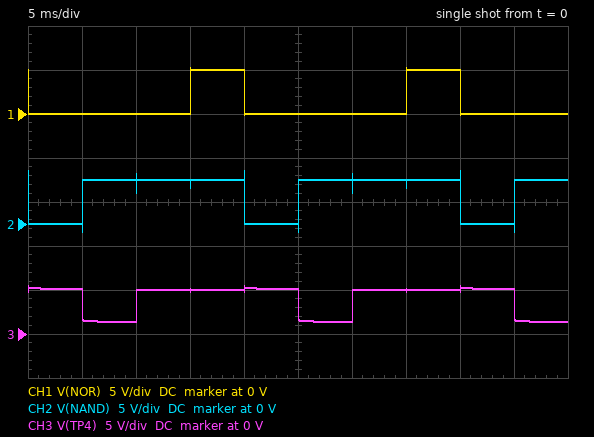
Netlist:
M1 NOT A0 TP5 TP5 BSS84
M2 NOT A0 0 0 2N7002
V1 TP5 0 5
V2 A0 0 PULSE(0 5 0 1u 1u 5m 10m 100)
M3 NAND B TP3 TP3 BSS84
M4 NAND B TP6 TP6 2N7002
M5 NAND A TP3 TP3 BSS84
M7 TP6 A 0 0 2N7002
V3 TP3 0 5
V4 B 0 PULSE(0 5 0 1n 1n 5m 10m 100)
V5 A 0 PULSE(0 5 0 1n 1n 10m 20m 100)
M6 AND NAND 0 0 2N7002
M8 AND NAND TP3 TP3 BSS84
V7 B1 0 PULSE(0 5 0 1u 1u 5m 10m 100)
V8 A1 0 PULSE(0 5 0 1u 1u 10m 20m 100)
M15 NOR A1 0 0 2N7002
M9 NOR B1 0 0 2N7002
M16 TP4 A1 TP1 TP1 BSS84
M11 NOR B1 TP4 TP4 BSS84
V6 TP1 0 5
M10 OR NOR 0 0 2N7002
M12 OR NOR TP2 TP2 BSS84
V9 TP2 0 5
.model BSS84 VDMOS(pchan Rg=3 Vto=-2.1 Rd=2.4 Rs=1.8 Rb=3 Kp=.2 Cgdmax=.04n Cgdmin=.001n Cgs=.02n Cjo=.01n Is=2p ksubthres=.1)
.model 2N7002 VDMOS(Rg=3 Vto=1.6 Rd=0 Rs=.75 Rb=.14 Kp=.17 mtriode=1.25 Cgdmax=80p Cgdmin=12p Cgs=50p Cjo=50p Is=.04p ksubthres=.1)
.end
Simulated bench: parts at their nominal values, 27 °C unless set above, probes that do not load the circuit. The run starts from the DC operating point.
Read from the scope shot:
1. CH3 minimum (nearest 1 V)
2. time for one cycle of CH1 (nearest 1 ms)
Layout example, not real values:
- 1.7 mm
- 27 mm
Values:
- 1 V
- 20 ms
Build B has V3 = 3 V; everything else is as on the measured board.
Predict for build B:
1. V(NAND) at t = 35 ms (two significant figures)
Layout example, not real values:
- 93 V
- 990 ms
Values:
- 3.0 V
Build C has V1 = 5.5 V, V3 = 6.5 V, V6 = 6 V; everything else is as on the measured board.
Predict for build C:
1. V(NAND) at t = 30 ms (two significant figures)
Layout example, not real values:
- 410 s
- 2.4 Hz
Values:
- 6.5 V
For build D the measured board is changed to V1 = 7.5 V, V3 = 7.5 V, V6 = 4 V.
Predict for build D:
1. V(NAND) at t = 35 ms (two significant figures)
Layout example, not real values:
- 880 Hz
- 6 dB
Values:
- 7.5 V
